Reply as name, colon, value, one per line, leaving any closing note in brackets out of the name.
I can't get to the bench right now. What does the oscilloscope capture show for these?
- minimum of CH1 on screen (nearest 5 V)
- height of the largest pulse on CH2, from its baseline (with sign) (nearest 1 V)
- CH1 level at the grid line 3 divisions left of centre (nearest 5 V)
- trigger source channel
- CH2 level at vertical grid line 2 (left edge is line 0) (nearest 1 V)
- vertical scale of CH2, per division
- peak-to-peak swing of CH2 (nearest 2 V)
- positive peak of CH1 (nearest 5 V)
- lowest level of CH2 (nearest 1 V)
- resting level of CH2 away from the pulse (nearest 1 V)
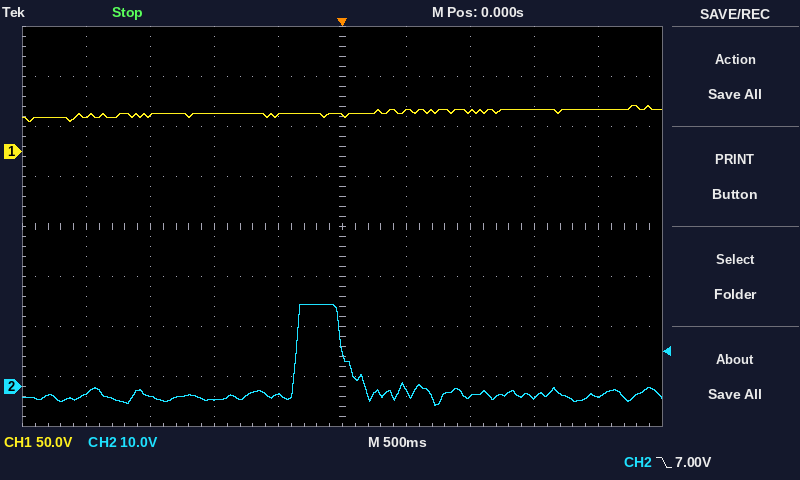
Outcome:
minimum of CH1 on screen: 30 V
height of the largest pulse on CH2, from its baseline (with sign): +18 V
CH1 level at the grid line 3 divisions left of centre: 35 V
trigger source channel: CH2
CH2 level at vertical grid line 2 (left edge is line 0): -2 V
vertical scale of CH2, per division: 10 V
peak-to-peak swing of CH2: 20 V
positive peak of CH1: 45 V
lowest level of CH2: -4 V
resting level of CH2 away from the pulse: -2 V
